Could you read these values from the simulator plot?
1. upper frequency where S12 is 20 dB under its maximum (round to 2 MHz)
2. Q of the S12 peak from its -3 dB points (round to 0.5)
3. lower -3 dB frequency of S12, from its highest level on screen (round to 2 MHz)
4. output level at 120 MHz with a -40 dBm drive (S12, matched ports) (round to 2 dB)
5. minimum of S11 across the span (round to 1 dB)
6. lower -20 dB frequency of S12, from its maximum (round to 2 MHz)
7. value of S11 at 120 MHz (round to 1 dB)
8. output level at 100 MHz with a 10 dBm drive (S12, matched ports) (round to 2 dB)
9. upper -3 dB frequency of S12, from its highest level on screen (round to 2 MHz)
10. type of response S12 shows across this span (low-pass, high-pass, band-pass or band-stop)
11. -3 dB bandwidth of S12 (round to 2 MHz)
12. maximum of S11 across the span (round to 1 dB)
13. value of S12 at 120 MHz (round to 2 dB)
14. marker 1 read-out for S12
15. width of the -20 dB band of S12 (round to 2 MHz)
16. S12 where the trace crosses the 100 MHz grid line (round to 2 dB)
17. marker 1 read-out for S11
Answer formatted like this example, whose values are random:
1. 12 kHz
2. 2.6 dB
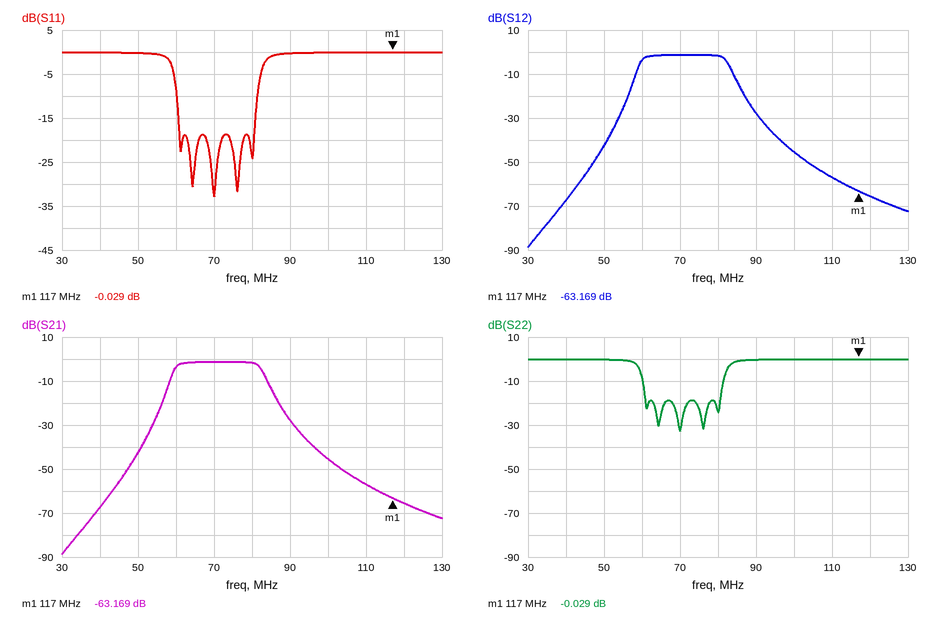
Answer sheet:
1. 88 MHz
2. 3.0
3. 60 MHz
4. -106 dBm
5. -33 dB
6. 56 MHz
7. 0 dB
8. -36 dBm
9. 82 MHz
10. band-pass
11. 22 MHz
12. 0 dB
13. -66 dB
14. -63.169 dB
15. 32 MHz
16. -46 dB
17. -0.029 dB
